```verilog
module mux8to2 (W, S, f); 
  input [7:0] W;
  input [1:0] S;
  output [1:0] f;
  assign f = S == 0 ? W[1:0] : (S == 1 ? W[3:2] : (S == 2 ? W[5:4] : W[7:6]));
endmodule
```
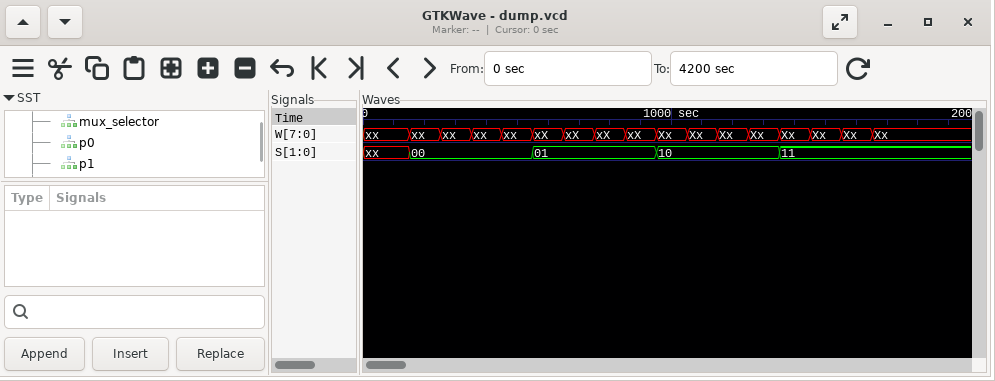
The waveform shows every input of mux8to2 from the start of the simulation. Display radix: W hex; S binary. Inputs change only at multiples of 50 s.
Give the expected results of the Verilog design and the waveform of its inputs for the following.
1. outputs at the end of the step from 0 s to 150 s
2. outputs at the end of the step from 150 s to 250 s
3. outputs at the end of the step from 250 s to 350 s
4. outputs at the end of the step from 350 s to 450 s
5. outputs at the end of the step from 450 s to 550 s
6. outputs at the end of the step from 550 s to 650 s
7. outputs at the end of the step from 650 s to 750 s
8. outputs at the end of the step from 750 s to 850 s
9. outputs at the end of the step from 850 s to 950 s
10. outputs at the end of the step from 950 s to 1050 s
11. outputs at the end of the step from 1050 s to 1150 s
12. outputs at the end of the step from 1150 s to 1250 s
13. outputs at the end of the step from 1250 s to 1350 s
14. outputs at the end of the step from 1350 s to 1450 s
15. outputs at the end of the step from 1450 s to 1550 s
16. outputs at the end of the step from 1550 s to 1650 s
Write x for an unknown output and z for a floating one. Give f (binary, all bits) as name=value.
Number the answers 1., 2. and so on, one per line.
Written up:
1. f=x
2. f=00
3. f=01
4. f=10
5. f=11
6. f=00
7. f=01
8. f=10
9. f=11
10. f=00
11. f=01
12. f=10
13. f=11
14. f=00
15. f=01
16. f=10
